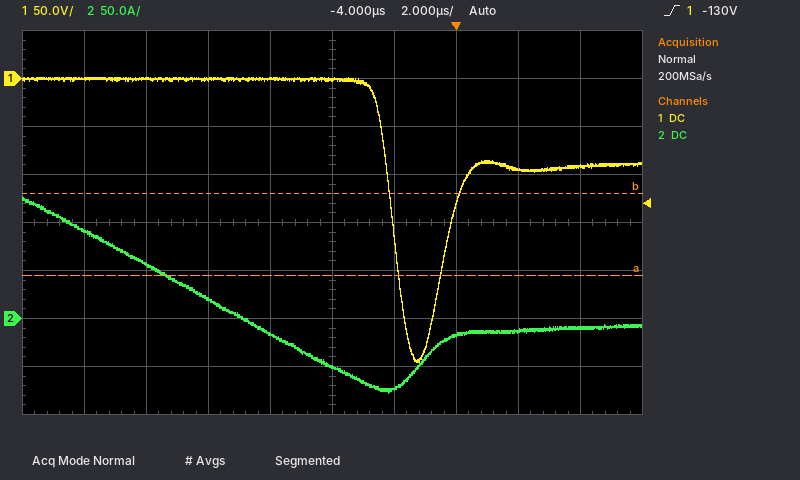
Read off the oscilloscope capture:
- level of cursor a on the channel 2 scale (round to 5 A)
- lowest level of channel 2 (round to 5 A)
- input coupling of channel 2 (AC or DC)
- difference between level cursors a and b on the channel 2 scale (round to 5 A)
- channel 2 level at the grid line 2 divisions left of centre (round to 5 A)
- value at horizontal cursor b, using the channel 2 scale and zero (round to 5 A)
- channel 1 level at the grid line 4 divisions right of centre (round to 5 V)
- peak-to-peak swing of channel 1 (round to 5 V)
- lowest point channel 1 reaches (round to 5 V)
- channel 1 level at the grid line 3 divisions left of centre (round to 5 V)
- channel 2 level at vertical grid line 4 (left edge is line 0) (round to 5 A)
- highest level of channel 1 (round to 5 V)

45 A
-75 A
DC
85 A
20 A
130 A
-90 V
295 V
-295 V
0 V
-15 A
0 V
